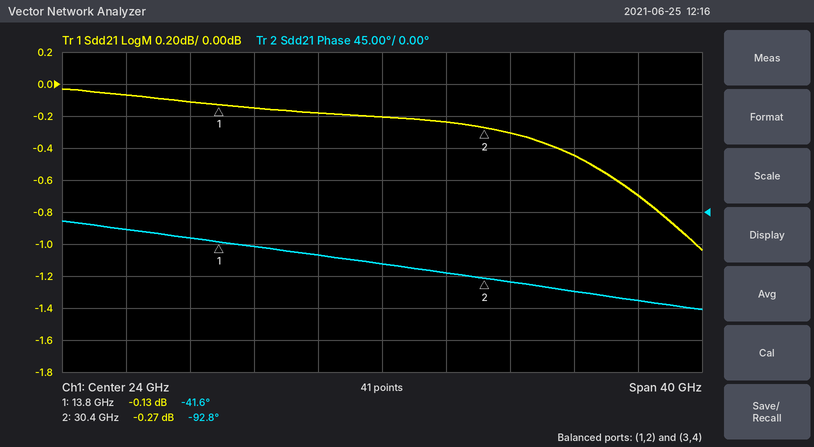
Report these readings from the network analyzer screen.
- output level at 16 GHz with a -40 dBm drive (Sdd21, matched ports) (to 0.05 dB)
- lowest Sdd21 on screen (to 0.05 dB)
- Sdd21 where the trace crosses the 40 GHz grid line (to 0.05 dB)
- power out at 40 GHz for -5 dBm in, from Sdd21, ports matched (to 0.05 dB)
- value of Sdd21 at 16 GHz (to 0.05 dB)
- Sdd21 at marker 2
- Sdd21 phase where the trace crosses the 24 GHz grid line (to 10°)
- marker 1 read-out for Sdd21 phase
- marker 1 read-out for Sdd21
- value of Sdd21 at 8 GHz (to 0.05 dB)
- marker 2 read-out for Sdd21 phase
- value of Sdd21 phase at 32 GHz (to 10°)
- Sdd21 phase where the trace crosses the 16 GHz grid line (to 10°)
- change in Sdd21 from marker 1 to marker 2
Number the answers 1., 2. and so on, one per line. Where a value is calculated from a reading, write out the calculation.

1. -40 dBm + (-0.15 dB) = -40.15 dBm
2. -1.05 dB
3. -0.70 dB
4. -5 dBm + (-0.70 dB) = -5.70 dBm
5. -0.15 dB
6. -0.27 dB
7. -70°
8. -41.6°
9. -0.13 dB
10. -0.05 dB
11. -92.8°
12. -100°
13. -50°
14. -0.27 − (-0.13) = -0.14 dB
